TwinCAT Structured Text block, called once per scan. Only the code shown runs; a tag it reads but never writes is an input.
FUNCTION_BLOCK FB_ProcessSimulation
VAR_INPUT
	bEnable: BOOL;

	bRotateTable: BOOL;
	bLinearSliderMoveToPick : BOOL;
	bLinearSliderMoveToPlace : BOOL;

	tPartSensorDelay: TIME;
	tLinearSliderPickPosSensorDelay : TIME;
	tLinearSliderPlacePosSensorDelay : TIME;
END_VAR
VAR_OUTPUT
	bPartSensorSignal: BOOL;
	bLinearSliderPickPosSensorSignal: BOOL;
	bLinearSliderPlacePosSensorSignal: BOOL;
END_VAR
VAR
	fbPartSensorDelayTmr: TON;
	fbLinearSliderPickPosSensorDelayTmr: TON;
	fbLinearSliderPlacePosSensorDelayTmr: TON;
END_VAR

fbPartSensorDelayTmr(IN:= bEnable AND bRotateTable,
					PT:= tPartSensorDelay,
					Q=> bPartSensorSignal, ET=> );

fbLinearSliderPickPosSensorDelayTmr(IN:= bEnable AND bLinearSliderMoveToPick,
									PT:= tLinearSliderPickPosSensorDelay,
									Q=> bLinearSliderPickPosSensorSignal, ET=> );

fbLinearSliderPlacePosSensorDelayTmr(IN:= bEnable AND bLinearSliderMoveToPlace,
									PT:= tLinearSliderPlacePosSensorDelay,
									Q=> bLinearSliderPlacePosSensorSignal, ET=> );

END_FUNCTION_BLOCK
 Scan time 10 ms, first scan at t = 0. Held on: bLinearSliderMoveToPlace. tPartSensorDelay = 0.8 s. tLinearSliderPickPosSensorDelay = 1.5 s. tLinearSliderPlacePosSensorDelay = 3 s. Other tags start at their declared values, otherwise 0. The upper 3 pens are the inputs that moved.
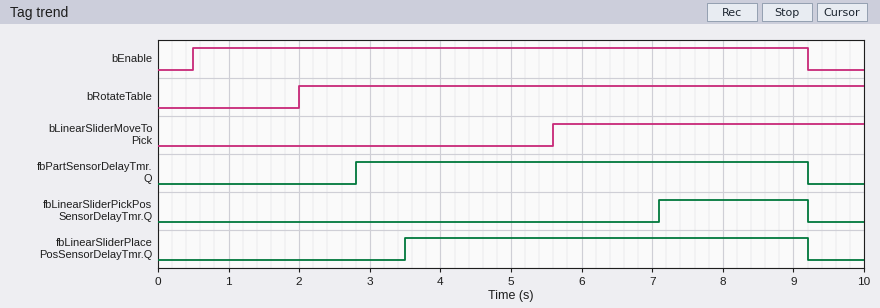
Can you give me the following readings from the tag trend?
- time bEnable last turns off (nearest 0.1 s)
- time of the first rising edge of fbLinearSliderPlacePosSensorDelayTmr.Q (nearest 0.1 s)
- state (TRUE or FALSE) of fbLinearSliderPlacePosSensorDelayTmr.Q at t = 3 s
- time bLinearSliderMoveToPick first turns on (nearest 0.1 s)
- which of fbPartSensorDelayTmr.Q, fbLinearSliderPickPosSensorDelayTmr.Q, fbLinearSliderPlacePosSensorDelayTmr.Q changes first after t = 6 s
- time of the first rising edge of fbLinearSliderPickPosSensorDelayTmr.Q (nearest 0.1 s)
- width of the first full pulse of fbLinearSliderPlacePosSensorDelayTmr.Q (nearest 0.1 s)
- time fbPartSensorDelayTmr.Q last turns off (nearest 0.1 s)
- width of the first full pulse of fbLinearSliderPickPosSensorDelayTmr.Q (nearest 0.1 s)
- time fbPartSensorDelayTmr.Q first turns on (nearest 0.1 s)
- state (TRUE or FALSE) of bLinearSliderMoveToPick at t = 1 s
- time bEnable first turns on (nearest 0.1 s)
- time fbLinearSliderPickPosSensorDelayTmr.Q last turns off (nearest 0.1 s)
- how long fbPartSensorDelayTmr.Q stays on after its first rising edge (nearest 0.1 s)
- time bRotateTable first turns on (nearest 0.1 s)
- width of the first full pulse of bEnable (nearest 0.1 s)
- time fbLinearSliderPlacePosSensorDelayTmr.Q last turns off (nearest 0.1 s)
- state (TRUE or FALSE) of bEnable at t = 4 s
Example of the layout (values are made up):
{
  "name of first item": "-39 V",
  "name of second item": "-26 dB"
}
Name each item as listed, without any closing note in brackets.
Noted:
{
  "time bEnable last turns off": "9.2 s",
  "time of the first rising edge of fbLinearSliderPlacePosSensorDelayTmr.Q": "3.5 s",
  "state (TRUE or FALSE) of fbLinearSliderPlacePosSensorDelayTmr.Q at t = 3 s": "FALSE",
  "time bLinearSliderMoveToPick first turns on": "5.6 s",
  "which of fbPartSensorDelayTmr.Q, fbLinearSliderPickPosSensorDelayTmr.Q, fbLinearSliderPlacePosSensorDelayTmr.Q changes first after t = 6 s": "fbLinearSliderPickPosSensorDelayTmr.Q",
  "time of the first rising edge of fbLinearSliderPickPosSensorDelayTmr.Q": "7.1 s",
  "width of the first full pulse of fbLinearSliderPlacePosSensorDelayTmr.Q": "5.7 s",
  "time fbPartSensorDelayTmr.Q last turns off": "9.2 s",
  "width of the first full pulse of fbLinearSliderPickPosSensorDelayTmr.Q": "2.1 s",
  "time fbPartSensorDelayTmr.Q first turns on": "2.8 s",
  "state (TRUE or FALSE) of bLinearSliderMoveToPick at t = 1 s": "FALSE",
  "time bEnable first turns on": "0.5 s",
  "time fbLinearSliderPickPosSensorDelayTmr.Q last turns off": "9.2 s",
  "how long fbPartSensorDelayTmr.Q stays on after its first rising edge": "6.4 s",
  "time bRotateTable first turns on": "2.0 s",
  "width of the first full pulse of bEnable": "8.7 s",
  "time fbLinearSliderPlacePosSensorDelayTmr.Q last turns off": "9.2 s",
  "state (TRUE or FALSE) of bEnable at t = 4 s": "TRUE"
}
